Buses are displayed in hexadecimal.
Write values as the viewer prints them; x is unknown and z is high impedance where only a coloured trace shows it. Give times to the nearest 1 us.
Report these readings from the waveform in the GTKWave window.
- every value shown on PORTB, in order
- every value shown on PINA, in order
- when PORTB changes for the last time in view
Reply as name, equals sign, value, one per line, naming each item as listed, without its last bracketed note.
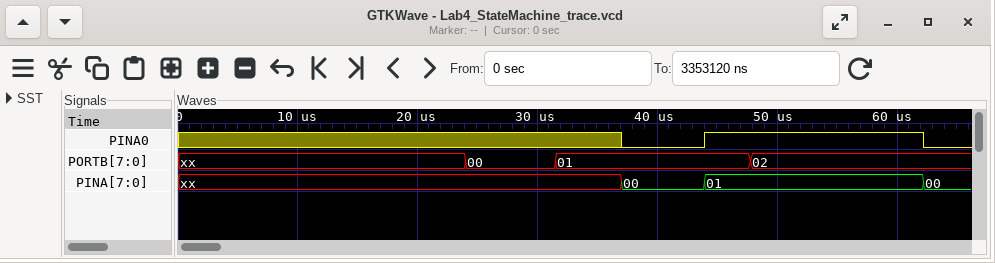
every value shown on PORTB, in order = xx, 00, 01, 02
every value shown on PINA, in order = xx, 00, 01, 00
when PORTB changes for the last time in view = 48 us
